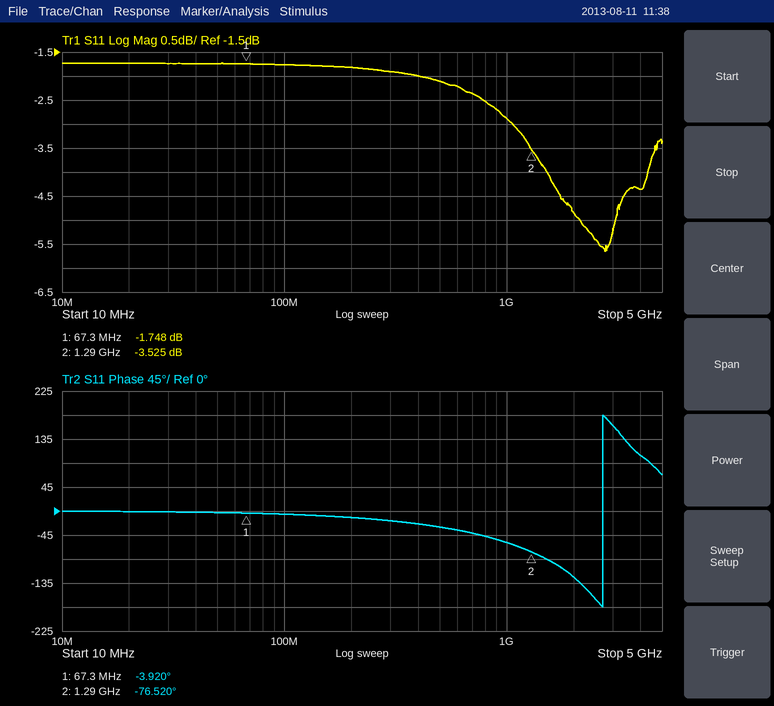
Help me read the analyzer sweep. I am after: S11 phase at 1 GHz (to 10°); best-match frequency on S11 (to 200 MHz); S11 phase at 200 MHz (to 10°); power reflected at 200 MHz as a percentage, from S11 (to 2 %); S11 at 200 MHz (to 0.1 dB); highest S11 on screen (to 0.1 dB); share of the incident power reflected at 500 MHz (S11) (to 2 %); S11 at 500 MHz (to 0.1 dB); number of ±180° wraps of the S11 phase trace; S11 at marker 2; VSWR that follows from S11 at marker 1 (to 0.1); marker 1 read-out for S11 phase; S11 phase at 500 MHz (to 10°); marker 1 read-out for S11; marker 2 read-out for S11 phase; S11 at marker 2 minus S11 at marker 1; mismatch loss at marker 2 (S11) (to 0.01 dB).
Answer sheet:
-60°
2.8 GHz
-10°
66 %
-1.8 dB
-1.7 dB
62 %
-2.1 dB
1
-3.525 dB
10.0
-3.920°
-30°
-1.748 dB
-76.520°
-1.777 dB
2.55 dB
